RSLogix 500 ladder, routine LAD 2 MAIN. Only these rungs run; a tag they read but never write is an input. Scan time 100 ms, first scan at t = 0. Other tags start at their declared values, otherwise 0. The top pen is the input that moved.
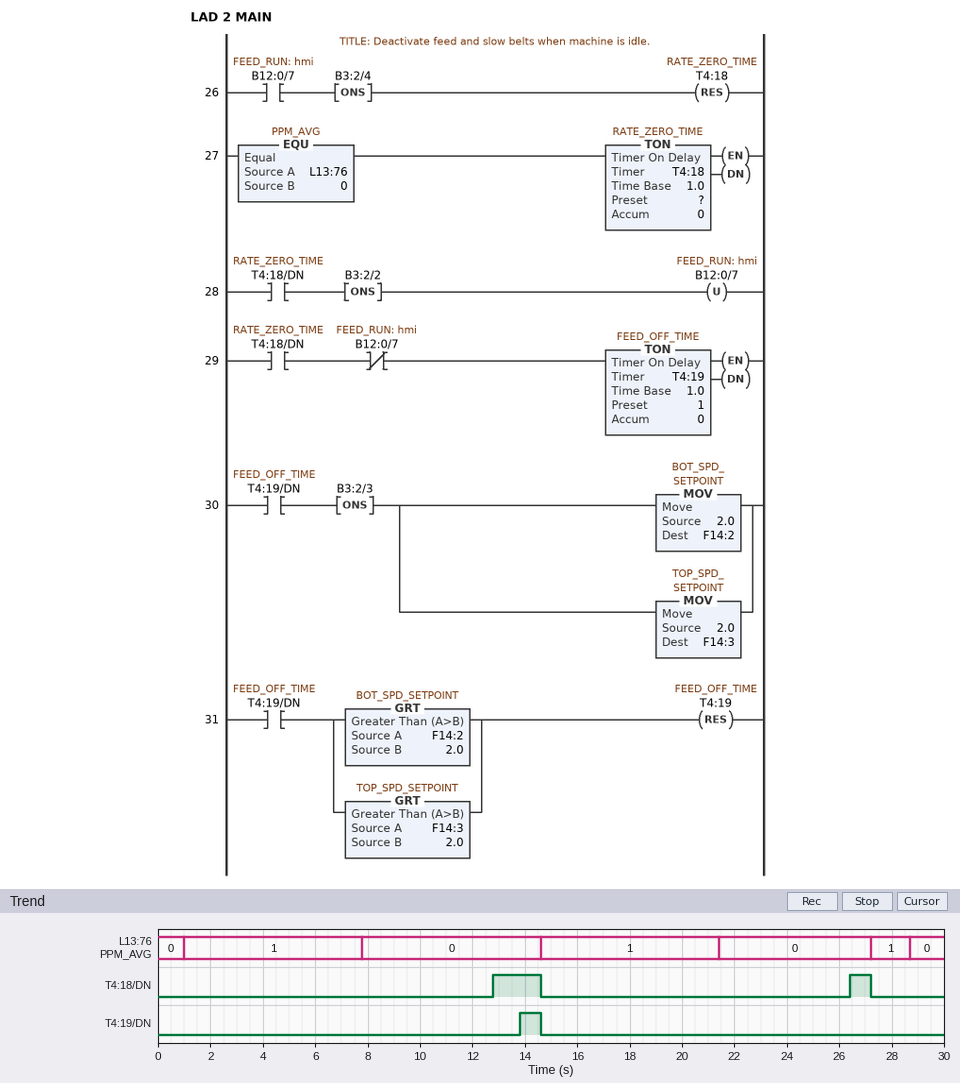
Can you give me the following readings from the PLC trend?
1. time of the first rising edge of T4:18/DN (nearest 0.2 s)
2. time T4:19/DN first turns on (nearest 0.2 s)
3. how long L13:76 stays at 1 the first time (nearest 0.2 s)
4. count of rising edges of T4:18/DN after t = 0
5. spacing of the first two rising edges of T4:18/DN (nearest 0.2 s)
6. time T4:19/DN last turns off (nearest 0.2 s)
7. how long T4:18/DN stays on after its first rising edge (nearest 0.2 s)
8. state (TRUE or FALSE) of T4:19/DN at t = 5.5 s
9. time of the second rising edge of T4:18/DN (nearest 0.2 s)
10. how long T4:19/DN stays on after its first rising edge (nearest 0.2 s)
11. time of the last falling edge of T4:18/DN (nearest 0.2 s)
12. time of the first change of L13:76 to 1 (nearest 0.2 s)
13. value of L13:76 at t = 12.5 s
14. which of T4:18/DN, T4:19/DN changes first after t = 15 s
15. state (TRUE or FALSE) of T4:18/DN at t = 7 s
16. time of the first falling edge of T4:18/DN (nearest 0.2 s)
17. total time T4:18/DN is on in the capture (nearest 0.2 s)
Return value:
12.8 s
13.8 s
6.8 s
2
13.6 s
14.6 s
1.8 s
FALSE
26.4 s
0.8 s
27.2 s
1.0 s
0
T4:18/DN
FALSE
14.6 s
2.6 s
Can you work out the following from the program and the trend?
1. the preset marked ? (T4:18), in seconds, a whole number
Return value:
5 s
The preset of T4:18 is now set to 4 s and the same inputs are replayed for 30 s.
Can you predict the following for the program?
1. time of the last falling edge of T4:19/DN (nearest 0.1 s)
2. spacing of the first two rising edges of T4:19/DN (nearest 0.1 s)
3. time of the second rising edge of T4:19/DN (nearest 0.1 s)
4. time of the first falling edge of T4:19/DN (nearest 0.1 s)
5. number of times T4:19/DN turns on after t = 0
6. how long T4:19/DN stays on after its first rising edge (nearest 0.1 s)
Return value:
27.2 s
13.6 s
26.4 s
14.6 s
2
1.8 s
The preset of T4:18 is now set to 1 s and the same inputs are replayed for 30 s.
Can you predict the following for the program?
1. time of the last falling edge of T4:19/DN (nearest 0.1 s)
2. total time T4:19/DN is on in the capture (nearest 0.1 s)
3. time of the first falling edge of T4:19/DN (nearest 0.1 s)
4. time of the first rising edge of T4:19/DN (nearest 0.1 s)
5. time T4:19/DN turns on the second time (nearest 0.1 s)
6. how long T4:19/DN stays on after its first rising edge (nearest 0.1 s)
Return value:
27.2 s
8.6 s
14.6 s
9.8 s
23.4 s
4.8 s
